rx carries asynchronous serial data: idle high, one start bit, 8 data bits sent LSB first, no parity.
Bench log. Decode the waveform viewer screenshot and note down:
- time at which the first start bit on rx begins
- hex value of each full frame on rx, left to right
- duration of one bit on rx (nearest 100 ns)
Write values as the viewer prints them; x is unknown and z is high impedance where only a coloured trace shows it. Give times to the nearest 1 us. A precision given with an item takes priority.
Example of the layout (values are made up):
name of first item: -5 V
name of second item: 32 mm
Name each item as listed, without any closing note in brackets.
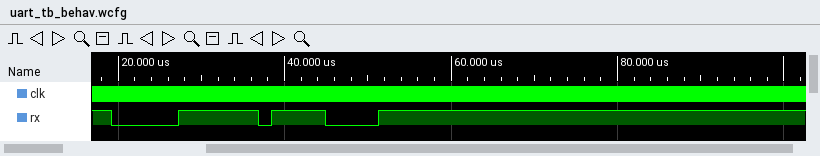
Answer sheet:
time at which the first start bit on rx begins: 19 us
hex value of each full frame on rx, left to right: F0, 0F
duration of one bit on rx: 1600 ns
